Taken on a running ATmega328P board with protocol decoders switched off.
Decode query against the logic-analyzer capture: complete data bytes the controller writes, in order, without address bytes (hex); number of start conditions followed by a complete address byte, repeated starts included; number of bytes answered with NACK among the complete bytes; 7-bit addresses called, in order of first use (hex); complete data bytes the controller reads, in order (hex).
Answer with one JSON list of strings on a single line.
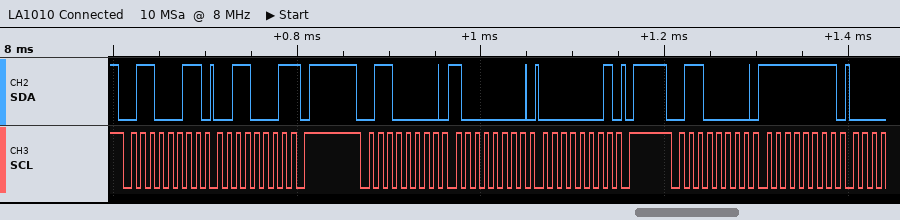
["80 01 FF", "3", "1", "0x31 0x30", "31"]
